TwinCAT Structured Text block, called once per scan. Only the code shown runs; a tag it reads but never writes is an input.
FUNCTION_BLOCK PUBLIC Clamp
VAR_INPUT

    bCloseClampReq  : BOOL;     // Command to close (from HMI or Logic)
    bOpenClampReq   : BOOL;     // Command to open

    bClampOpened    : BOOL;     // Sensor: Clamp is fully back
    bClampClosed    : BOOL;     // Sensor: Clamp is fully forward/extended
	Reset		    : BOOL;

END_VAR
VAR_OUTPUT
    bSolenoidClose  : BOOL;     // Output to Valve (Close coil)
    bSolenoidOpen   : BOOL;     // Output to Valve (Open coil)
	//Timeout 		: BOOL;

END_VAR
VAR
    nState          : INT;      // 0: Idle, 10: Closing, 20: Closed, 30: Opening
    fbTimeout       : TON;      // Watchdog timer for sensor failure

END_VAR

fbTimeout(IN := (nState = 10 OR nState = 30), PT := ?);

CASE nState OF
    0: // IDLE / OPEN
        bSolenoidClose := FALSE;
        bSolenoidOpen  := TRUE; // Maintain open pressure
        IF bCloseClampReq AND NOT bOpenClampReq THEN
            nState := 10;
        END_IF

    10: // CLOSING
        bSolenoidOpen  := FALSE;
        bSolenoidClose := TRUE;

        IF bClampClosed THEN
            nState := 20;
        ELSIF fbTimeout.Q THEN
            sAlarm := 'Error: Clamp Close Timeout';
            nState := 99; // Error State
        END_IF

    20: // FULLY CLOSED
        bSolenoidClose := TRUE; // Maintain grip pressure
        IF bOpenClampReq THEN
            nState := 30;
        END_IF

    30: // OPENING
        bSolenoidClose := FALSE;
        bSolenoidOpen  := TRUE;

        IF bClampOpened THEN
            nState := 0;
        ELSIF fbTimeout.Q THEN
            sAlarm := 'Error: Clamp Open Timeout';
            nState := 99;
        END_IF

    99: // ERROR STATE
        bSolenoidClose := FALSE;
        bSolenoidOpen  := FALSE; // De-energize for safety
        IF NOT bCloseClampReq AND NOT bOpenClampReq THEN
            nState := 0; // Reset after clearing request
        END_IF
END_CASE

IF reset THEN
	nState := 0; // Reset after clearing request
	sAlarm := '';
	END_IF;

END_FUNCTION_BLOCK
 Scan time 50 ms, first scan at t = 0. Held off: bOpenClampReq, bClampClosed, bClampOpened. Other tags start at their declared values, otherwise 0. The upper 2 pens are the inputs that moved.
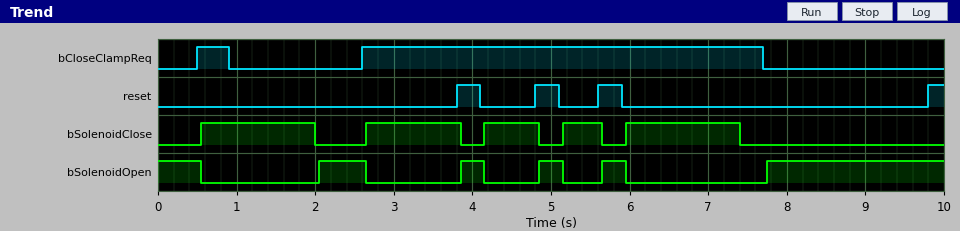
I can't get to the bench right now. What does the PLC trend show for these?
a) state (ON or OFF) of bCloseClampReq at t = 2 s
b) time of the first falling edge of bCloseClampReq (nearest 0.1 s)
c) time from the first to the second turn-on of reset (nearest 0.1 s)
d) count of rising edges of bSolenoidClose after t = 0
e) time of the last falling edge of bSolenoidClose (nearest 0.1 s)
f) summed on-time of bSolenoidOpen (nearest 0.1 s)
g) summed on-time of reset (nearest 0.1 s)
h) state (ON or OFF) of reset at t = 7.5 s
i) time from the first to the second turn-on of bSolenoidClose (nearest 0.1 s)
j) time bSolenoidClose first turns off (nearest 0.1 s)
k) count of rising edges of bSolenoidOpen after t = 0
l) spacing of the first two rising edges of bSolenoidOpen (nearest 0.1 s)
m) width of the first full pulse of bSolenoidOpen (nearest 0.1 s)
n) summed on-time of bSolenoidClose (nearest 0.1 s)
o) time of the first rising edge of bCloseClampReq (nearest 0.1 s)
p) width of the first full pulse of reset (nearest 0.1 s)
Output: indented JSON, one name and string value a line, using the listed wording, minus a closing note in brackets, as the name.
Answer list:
{
  "state (ON or OFF) of bCloseClampReq at t = 2 s": "OFF",
  "time of the first falling edge of bCloseClampReq": "0.9 s",
  "time from the first to the second turn-on of reset": "1.0 s",
  "count of rising edges of bSolenoidClose after t = 0": "5",
  "time of the last falling edge of bSolenoidClose": "7.4 s",
  "summed on-time of bSolenoidOpen": "4.3 s",
  "summed on-time of reset": "1.1 s",
  "state (ON or OFF) of reset at t = 7.5 s": "OFF",
  "time from the first to the second turn-on of bSolenoidClose": "2.1 s",
  "time bSolenoidClose first turns off": "2.0 s",
  "count of rising edges of bSolenoidOpen after t = 0": "5",
  "spacing of the first two rising edges of bSolenoidOpen": "1.8 s",
  "width of the first full pulse of bSolenoidOpen": "0.6 s",
  "summed on-time of bSolenoidClose": "5.3 s",
  "time of the first rising edge of bCloseClampReq": "0.5 s",
  "width of the first full pulse of reset": "0.3 s"
}
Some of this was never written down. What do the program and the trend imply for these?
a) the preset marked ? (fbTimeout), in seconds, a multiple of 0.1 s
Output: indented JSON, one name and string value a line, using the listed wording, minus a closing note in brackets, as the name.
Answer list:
{
  "the preset marked ? (fbTimeout), in seconds, a multiple of 0.1 s": "1.4 s"
}
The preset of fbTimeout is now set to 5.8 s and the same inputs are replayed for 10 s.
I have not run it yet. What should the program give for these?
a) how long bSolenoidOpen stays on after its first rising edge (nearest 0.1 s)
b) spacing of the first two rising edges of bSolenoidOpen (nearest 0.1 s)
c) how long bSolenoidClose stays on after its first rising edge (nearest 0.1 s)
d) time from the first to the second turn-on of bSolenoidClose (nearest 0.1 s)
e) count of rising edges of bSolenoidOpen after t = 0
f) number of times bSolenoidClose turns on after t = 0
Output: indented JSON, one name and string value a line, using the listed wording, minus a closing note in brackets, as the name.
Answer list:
{
  "how long bSolenoidOpen stays on after its first rising edge": "0.3 s",
  "spacing of the first two rising edges of bSolenoidOpen": "1.0 s",
  "how long bSolenoidClose stays on after its first rising edge": "3.3 s",
  "time from the first to the second turn-on of bSolenoidClose": "3.6 s",
  "count of rising edges of bSolenoidOpen after t = 0": "4",
  "number of times bSolenoidClose turns on after t = 0": "4"
}
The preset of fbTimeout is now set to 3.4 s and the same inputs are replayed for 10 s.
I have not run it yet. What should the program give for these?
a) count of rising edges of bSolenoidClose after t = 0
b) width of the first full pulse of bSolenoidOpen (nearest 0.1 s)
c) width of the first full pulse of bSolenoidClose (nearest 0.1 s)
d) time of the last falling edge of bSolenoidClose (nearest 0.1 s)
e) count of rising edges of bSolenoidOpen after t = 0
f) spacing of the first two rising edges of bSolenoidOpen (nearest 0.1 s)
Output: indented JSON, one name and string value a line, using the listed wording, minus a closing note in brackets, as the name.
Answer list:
{
  "count of rising edges of bSolenoidClose after t = 0": "4",
  "width of the first full pulse of bSolenoidOpen": "0.3 s",
  "width of the first full pulse of bSolenoidClose": "3.3 s",
  "time of the last falling edge of bSolenoidClose": "9.4 s",
  "count of rising edges of bSolenoidOpen after t = 0": "4",
  "spacing of the first two rising edges of bSolenoidOpen": "1.0 s"
}
